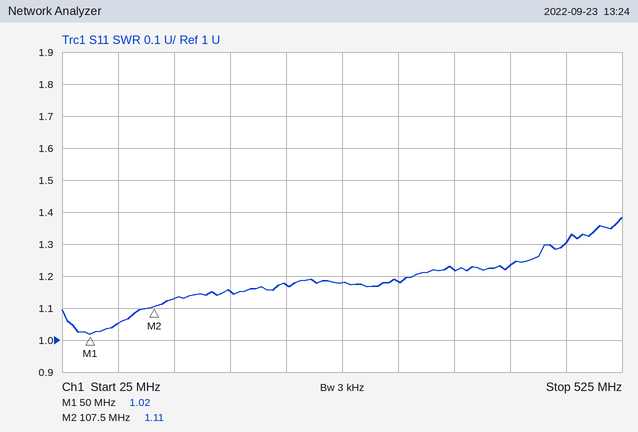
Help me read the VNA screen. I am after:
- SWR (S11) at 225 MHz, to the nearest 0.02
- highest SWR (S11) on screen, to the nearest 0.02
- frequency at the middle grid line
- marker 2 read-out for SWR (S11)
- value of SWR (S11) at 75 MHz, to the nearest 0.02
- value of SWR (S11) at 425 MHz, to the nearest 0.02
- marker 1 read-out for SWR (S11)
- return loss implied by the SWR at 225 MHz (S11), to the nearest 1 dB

1.18
1.38
275 MHz
1.11
1.06
1.24
1.02
22 dB
